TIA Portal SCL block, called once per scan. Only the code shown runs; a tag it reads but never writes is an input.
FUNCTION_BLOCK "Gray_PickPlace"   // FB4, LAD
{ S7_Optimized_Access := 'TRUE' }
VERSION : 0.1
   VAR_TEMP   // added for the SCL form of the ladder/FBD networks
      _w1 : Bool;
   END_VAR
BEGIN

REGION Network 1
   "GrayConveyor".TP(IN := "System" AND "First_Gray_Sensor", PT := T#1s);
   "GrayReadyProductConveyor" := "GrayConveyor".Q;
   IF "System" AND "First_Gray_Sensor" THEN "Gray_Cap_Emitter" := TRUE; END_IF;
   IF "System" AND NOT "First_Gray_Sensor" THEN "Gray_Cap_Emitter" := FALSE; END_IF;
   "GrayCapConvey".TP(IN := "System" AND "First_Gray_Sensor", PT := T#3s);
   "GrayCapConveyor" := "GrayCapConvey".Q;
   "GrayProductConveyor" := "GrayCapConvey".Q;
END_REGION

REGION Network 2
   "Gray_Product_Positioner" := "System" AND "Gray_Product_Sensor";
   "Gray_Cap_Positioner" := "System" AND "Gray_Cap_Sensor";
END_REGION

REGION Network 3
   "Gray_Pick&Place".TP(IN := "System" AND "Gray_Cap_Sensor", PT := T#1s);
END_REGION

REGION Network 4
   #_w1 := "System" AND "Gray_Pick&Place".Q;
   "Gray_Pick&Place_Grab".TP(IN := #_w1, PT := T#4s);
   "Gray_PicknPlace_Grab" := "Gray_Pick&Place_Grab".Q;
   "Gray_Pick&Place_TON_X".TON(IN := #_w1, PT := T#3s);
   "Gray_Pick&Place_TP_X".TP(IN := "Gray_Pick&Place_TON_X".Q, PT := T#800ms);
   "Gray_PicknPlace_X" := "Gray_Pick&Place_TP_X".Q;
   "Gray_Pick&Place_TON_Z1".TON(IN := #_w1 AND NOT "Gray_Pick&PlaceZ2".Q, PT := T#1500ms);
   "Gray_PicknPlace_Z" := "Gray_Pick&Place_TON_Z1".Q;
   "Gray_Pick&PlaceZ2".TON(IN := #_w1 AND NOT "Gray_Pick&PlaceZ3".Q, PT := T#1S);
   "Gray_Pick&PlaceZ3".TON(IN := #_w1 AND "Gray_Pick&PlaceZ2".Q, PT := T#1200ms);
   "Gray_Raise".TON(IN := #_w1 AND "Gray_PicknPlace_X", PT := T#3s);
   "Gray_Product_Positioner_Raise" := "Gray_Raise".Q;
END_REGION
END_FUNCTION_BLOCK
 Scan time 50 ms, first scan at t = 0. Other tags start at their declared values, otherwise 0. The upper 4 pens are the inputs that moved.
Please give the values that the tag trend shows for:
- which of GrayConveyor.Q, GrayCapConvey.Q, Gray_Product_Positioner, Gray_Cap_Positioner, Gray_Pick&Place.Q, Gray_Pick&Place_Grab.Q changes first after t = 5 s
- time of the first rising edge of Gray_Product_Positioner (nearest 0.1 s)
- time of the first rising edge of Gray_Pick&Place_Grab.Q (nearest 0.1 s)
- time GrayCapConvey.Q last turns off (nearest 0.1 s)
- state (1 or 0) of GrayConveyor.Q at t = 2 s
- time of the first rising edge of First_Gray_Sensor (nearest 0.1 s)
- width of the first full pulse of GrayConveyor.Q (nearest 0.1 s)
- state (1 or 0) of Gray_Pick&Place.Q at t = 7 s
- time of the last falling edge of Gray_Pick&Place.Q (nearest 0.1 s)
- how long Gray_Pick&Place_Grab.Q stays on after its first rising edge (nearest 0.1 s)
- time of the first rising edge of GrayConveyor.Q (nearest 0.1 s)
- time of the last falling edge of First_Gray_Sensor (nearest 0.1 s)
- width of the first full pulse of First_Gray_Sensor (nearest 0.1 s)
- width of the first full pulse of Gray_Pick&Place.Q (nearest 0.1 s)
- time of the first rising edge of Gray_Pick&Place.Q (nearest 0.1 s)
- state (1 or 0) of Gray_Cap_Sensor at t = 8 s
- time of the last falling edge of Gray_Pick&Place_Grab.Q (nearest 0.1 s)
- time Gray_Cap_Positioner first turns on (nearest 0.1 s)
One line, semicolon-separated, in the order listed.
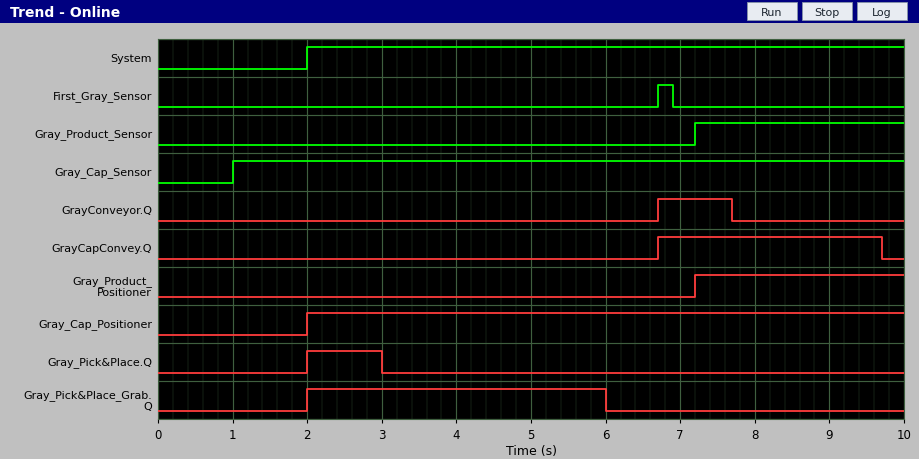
Gray_Pick&Place_Grab.Q; 7.2 s; 2.0 s; 9.7 s; 0; 6.7 s; 1.0 s; 0; 3.0 s; 4.0 s; 6.7 s; 6.9 s; 0.2 s; 1.0 s; 2.0 s; 1; 6.0 s; 2.0 s
